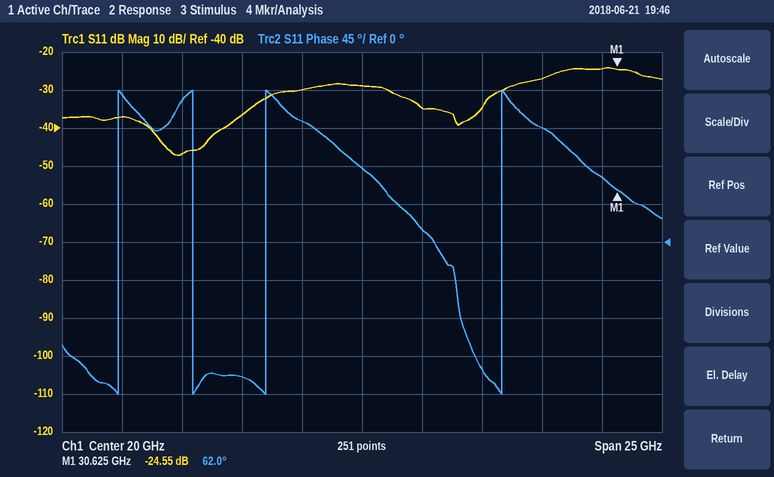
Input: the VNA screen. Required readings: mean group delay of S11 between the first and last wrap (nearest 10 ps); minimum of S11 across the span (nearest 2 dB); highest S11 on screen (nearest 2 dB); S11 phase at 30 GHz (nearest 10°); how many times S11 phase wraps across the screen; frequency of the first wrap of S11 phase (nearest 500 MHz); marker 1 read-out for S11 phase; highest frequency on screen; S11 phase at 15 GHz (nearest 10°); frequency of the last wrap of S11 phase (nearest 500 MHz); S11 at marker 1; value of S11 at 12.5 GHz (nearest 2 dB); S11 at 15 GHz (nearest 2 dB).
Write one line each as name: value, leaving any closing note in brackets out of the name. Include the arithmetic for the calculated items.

mean group delay of S11 between the first and last wrap: 3 cycles / (26.0 GHz − 10.0 GHz) ≈ 188 ps, so 190 ps to the nearest 10 ps
minimum of S11 across the span: -48 dB
highest S11 on screen: -24 dB
S11 phase at 30 GHz: 80°
how many times S11 phase wraps across the screen: 4
frequency of the first wrap of S11 phase: 10.0 GHz
marker 1 read-out for S11 phase: 62.0°
highest frequency on screen: 32.5 GHz
S11 phase at 15 GHz: -160°
frequency of the last wrap of S11 phase: 26.0 GHz
S11 at marker 1: -24.55 dB
value of S11 at 12.5 GHz: -46 dB
S11 at 15 GHz: -36 dB
